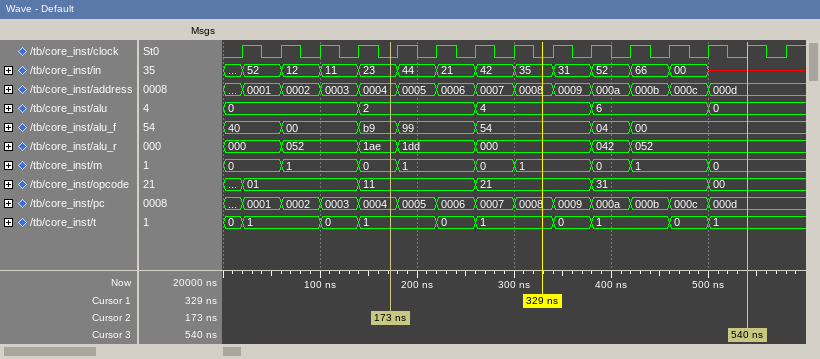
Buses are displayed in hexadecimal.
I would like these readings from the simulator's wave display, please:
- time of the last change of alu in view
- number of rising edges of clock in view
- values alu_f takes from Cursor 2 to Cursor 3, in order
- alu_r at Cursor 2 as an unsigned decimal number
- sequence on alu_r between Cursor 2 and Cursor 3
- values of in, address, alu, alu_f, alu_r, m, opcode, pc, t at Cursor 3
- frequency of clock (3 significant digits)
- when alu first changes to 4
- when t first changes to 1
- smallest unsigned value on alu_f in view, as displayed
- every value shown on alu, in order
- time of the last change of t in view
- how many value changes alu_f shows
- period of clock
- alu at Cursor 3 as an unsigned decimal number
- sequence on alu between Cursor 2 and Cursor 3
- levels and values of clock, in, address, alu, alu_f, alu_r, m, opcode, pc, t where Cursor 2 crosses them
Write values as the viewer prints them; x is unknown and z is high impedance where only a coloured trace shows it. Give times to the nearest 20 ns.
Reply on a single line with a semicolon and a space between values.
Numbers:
500 ns; 15; b9, 99, 54, 04, 00; 430; 1ae, 1dd, 000, 042, 052; in=x, address=000d, alu=0, alu_f=00, alu_r=052, m=0, opcode=00, pc=000d, t=1; 25.0 MHz; 260 ns; 20 ns; 00; 0, 2, 4, 6, 0; 500 ns; 6; 40 ns; 0; 2, 4, 6, 0; clock=0, in=23, address=0004, alu=2, alu_f=b9, alu_r=1ae, m=0, opcode=11, pc=0004, t=1
